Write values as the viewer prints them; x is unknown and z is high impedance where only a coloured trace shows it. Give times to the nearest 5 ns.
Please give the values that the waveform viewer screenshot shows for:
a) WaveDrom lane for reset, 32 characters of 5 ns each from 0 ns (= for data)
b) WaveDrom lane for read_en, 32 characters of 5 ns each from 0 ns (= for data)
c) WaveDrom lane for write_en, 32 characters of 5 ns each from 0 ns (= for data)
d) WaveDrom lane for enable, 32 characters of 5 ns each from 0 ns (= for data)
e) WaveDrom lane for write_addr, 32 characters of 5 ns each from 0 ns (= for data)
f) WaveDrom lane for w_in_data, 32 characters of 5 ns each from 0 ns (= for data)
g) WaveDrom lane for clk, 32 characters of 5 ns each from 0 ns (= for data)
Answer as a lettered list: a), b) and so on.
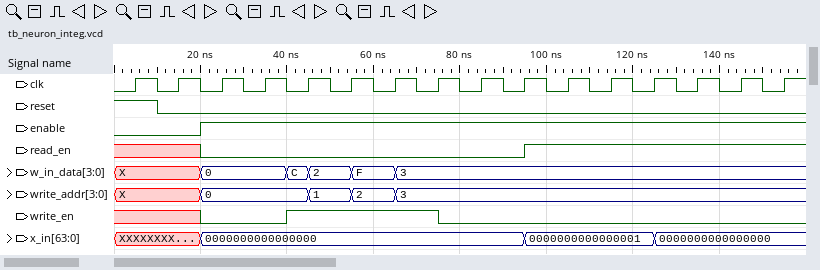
a) {name: 'reset', wave: '1.0.............................'}
b) {name: 'read_en', wave: 'x...0..............1............'}
c) {name: 'write_en', wave: 'x...0...1......0................'}
d) {name: 'enable', wave: '0...1...........................'}
e) {name: 'write_addr', wave: 'x...=....=.=.=..................', data: '0 1 2 3'}
f) {name: 'w_in_data', wave: 'x...=...==.=.=..................', data: '0 C 2 F 3'}
g) {name: 'clk', wave: '01010101010101010101010101010101'}
